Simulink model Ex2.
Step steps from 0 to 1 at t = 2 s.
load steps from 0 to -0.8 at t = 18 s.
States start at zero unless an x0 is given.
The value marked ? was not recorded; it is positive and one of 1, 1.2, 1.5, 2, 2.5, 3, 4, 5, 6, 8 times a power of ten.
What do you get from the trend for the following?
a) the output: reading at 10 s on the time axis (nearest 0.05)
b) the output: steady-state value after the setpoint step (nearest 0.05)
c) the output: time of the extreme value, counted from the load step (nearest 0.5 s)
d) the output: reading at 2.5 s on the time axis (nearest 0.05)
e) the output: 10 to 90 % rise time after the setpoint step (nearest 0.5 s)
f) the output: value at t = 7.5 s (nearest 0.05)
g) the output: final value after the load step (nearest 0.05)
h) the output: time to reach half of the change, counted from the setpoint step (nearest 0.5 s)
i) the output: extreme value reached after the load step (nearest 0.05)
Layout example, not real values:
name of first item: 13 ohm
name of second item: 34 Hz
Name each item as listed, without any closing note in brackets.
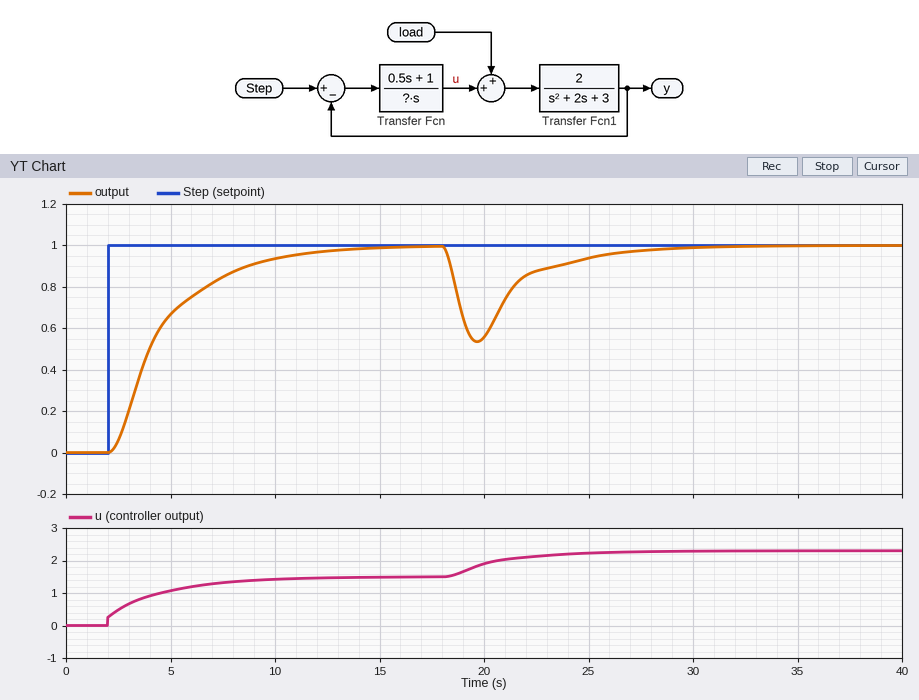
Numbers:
the output: reading at 10 s on the time axis: 0.95
the output: steady-state value after the setpoint step: 1.00
the output: time of the extreme value, counted from the load step: 1.5 s
the output: reading at 2.5 s on the time axis: 0.05
the output: 10 to 90 % rise time after the setpoint step: 6.0 s
the output: value at t = 7.5 s: 0.85
the output: final value after the load step: 1.00
the output: time to reach half of the change, counted from the setpoint step: 2.0 s
the output: extreme value reached after the load step: 0.55
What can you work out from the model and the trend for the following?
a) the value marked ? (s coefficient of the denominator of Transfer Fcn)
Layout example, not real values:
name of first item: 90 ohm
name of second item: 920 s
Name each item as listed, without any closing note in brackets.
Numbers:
the value marked ?: 2
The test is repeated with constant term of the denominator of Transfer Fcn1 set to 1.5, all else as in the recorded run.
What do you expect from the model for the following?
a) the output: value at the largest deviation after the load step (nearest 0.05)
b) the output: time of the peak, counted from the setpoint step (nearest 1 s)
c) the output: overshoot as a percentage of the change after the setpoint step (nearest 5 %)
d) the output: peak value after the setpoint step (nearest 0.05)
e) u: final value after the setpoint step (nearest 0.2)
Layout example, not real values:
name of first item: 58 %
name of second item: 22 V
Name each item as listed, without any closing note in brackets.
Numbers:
the output: value at the largest deviation after the load step: 0.35
the output: time of the peak, counted from the setpoint step: 4 s
the output: overshoot as a percentage of the change after the setpoint step: 10 %
the output: peak value after the setpoint step: 1.10
u: final value after the setpoint step: 0.8
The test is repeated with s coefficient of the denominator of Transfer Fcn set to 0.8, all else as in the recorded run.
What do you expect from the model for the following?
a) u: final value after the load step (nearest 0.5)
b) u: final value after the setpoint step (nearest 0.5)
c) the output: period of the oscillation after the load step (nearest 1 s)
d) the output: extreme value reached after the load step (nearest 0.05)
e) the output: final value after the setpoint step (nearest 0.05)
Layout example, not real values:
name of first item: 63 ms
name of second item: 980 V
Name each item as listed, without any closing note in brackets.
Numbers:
u: final value after the load step: 2.5
u: final value after the setpoint step: 1.5
the output: period of the oscillation after the load step: 4 s
the output: extreme value reached after the load step: 0.65
the output: final value after the setpoint step: 1.00
